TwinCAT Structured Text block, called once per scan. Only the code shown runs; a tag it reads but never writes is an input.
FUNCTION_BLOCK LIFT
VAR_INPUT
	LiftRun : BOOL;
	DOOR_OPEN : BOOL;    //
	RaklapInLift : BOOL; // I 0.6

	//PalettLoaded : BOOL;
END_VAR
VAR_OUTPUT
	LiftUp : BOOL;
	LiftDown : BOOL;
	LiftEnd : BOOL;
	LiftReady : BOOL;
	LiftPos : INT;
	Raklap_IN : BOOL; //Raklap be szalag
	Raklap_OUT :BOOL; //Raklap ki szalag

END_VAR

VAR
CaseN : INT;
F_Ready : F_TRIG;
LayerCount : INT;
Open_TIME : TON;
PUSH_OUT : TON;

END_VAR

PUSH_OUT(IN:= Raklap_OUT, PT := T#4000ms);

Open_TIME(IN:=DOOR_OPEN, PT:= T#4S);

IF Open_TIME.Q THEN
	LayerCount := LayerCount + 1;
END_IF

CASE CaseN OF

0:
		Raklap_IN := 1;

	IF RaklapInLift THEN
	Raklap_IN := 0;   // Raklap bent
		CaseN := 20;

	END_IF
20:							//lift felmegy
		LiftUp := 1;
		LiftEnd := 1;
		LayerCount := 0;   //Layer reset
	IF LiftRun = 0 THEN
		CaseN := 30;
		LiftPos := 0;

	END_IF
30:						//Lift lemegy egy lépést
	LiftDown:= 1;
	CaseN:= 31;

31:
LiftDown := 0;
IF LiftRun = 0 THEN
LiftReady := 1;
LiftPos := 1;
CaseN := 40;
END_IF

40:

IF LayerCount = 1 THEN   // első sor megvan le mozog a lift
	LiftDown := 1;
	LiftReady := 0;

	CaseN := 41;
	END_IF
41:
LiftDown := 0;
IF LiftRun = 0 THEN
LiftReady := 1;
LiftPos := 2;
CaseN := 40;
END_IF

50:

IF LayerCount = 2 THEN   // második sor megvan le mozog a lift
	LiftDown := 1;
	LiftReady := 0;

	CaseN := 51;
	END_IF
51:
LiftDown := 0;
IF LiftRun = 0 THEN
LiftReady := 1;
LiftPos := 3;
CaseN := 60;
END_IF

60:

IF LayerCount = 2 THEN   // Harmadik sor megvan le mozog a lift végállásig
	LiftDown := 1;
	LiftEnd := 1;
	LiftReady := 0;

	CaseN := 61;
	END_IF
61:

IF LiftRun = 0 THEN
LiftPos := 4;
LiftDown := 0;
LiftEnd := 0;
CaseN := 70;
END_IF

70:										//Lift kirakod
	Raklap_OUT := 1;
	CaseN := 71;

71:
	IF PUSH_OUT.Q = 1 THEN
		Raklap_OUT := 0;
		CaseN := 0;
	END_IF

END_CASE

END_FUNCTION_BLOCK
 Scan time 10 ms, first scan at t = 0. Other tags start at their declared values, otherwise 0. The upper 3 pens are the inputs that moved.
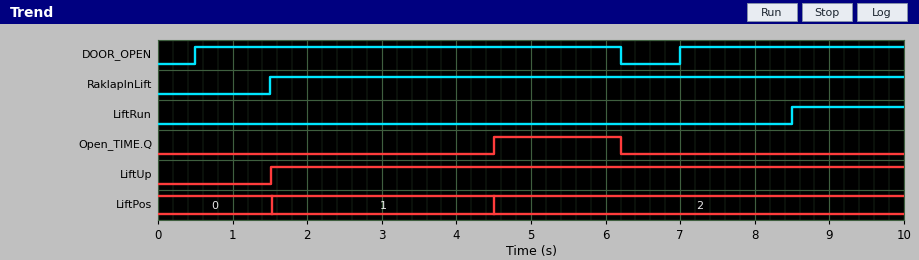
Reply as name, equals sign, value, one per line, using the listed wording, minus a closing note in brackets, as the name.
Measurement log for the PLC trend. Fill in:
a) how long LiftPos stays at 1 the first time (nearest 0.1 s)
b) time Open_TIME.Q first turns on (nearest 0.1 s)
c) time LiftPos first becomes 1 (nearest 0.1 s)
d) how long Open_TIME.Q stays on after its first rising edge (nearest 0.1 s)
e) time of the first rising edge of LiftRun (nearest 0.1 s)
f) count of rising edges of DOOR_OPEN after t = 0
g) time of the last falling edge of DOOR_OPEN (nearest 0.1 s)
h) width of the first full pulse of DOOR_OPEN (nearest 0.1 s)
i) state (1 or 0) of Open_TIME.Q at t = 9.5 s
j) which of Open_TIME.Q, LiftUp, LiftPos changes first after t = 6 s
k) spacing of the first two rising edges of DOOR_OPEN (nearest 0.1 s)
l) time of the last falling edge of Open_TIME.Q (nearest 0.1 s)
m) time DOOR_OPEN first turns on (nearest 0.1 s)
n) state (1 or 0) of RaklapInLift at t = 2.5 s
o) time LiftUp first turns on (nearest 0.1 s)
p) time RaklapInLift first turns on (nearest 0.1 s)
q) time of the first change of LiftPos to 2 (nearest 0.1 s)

how long LiftPos stays at 1 the first time = 3.0 s
time Open_TIME.Q first turns on = 4.5 s
time LiftPos first becomes 1 = 1.5 s
how long Open_TIME.Q stays on after its first rising edge = 1.7 s
time of the first rising edge of LiftRun = 8.5 s
count of rising edges of DOOR_OPEN after t = 0 = 2
time of the last falling edge of DOOR_OPEN = 6.2 s
width of the first full pulse of DOOR_OPEN = 5.7 s
state (1 or 0) of Open_TIME.Q at t = 9.5 s = 0
which of Open_TIME.Q, LiftUp, LiftPos changes first after t = 6 s = Open_TIME.Q
spacing of the first two rising edges of DOOR_OPEN = 6.5 s
time of the last falling edge of Open_TIME.Q = 6.2 s
time DOOR_OPEN first turns on = 0.5 s
state (1 or 0) of RaklapInLift at t = 2.5 s = 1
time LiftUp first turns on = 1.5 s
time RaklapInLift first turns on = 1.5 s
time of the first change of LiftPos to 2 = 4.5 s
